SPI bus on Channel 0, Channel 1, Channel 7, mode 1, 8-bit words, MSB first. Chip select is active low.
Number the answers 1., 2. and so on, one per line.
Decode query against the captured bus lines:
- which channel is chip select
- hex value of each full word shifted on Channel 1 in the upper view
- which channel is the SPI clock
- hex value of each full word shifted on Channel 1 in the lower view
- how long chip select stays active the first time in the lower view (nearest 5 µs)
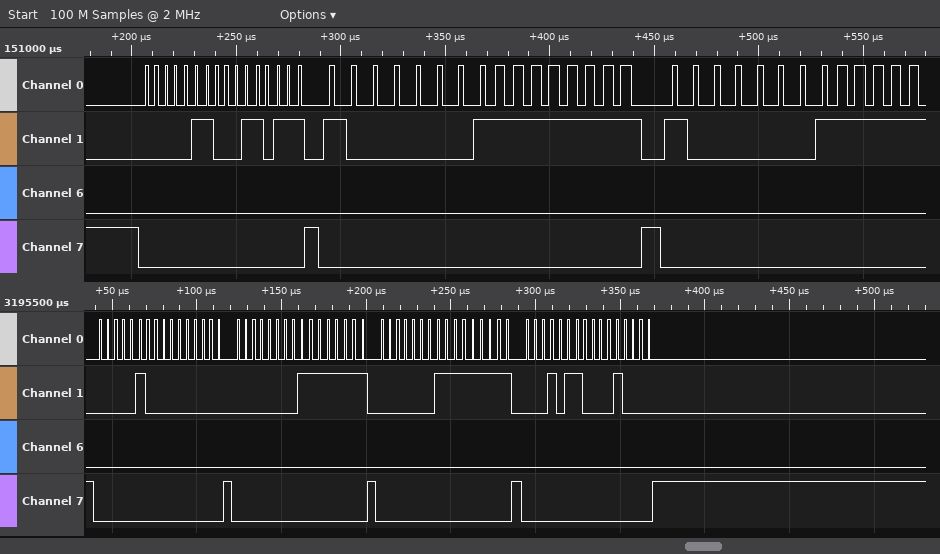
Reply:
1. Channel 7
2. 06, 37, 81, FF, 81
3. Channel 0
4. 04, 00, 00, FF, 01, FF, 16, 10
5. 75 µs
